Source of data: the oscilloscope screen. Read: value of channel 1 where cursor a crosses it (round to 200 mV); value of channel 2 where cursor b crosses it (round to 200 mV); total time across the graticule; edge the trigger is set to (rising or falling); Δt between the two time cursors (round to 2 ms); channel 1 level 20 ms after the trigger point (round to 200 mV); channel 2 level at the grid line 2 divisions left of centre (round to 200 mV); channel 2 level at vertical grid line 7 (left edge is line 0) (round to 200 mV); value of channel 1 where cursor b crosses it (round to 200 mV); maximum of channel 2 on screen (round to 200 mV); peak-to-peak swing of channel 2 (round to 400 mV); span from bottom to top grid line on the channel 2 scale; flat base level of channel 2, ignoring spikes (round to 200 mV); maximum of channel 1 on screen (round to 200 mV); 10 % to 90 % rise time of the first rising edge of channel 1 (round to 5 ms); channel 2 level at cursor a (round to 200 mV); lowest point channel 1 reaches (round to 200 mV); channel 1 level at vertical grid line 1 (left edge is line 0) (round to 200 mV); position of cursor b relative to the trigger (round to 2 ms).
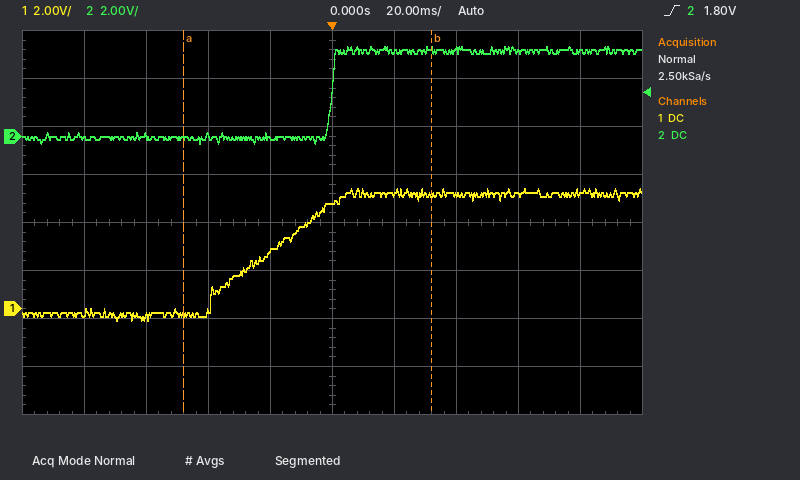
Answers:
-200 mV
3.6 V
200 ms
rising
80 ms
4.8 V
0.0 V
3.6 V
4.8 V
3.8 V
4.0 V
16 V
0.0 V
5.0 V
35 ms
0.0 V
-400 mV
-200 mV
+32 ms
